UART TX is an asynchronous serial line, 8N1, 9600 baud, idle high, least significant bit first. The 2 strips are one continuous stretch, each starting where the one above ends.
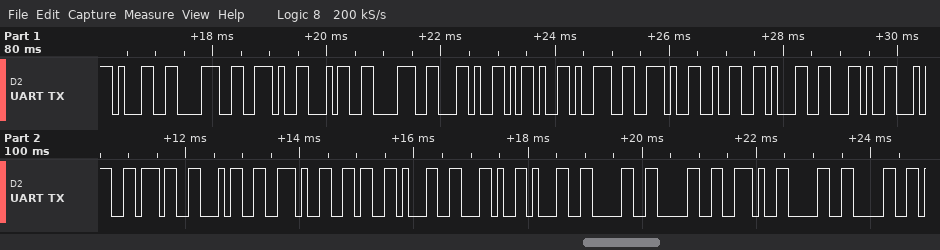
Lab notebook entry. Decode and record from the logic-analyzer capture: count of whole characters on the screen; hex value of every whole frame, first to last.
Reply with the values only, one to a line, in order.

25
31 38 2E 34 38 2C 2D 39 2E 32 31 2C 34 37 34 2E 36 31 2C 31 30 30 2E 30 30
